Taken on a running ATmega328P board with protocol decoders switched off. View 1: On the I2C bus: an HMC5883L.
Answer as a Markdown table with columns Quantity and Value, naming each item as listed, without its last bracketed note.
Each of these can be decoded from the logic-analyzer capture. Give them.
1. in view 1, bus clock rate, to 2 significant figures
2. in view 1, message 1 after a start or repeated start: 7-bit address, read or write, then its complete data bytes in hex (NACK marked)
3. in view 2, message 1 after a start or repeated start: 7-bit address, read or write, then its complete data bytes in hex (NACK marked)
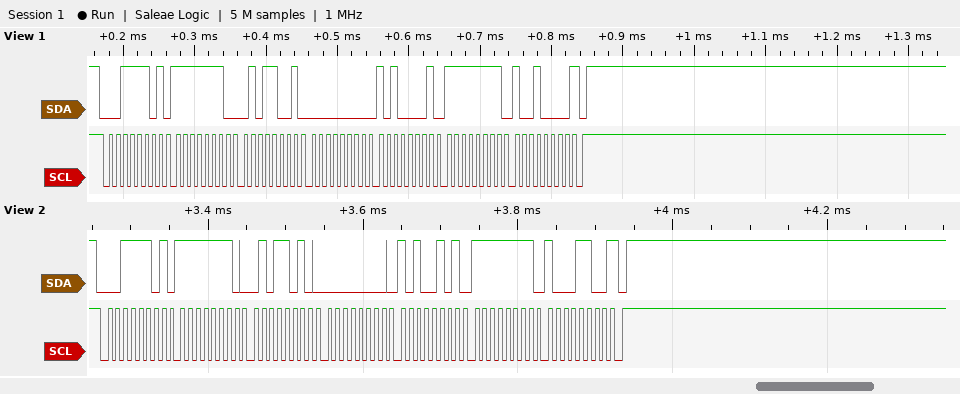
| Quantity | Value |
|---|---|
| in view 1, bus clock rate, to 2 significant figures | 100 kHz |
| in view 1, message 1 after a start or repeated start: 7-bit address, read or write, then its complete data bytes in hex | 0x1E read: FE 59 00 A1 FF 90 NACK |
| in view 2, message 1 after a start or repeated start: 7-bit address, read or write, then its complete data bytes in hex | 0x1E read: FE 5A 00 A5 FF 8C NACK |
